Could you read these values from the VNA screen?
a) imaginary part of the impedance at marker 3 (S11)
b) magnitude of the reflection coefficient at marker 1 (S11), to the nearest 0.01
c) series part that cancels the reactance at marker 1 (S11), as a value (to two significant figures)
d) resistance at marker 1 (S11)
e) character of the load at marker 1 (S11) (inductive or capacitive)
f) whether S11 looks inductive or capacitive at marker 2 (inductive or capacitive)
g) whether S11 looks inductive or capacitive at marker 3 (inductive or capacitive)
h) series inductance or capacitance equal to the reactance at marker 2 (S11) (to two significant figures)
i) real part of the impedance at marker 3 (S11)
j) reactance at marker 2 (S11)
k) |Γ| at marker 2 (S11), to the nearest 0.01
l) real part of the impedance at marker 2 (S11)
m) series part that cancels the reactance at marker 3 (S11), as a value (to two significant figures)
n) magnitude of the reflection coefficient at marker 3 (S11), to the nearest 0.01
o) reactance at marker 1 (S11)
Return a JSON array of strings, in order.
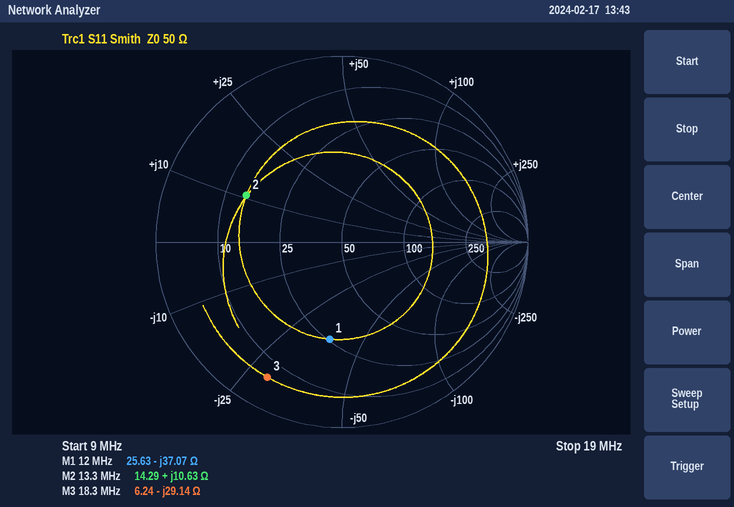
["-29.14 Ω", "0.53", "490 nH", "25.63 Ω", "capacitive", "inductive", "capacitive", "130 nH", "6.24 Ω", "+10.63 Ω", "0.57", "14.29 Ω", "250 nH", "0.83", "-37.07 Ω"]
